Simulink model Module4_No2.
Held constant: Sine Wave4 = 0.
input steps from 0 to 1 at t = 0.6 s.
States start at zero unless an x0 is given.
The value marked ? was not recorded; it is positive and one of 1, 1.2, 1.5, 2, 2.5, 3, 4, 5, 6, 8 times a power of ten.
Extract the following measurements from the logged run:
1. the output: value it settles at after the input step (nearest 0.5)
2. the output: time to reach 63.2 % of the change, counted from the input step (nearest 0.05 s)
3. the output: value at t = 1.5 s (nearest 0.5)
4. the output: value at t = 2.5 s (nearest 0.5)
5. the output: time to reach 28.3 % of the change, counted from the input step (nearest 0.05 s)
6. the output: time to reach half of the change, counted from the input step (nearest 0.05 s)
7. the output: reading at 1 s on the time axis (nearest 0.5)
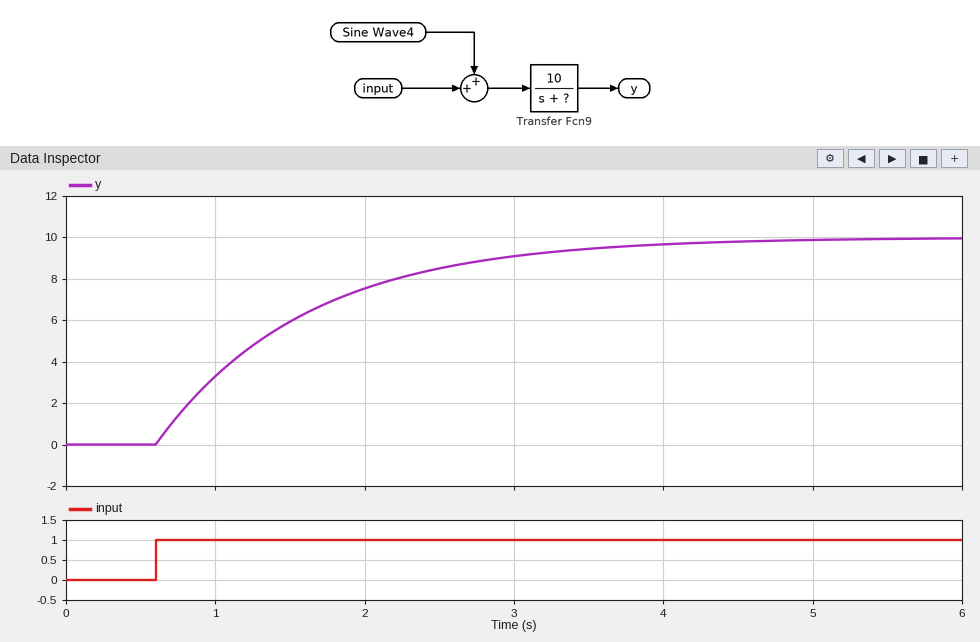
10.0
1.00 s
6.0
8.5
0.35 s
0.70 s
3.5
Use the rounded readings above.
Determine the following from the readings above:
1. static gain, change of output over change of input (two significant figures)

10
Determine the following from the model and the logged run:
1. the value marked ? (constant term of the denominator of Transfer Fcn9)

1
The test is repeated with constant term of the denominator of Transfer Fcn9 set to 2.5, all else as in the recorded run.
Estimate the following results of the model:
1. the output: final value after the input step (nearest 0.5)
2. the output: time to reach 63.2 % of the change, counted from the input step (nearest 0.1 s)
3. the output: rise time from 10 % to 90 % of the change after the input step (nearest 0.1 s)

4.0
0.4 s
0.9 s
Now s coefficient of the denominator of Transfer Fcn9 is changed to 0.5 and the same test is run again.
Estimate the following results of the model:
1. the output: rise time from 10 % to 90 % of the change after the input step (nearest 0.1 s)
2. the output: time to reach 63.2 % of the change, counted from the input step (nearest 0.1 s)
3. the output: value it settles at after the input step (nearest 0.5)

1.1 s
0.5 s
10.0
